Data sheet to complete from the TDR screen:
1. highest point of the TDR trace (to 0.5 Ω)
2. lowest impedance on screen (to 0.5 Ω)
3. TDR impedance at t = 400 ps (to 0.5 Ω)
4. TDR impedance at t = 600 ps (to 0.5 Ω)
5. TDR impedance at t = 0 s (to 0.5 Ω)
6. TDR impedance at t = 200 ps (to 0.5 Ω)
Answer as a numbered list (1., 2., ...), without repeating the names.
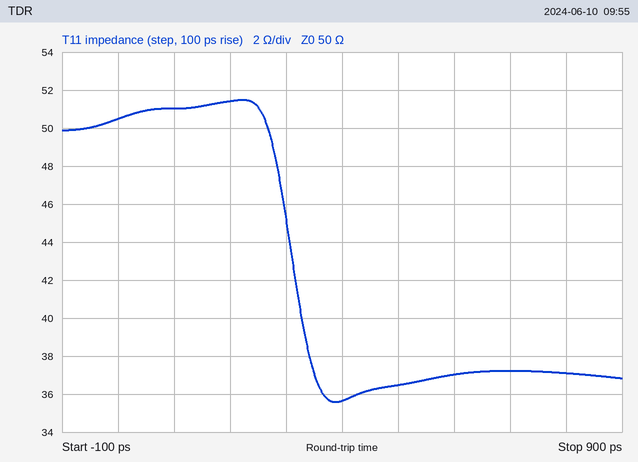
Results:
1. 51.5 Ω
2. 35.5 Ω
3. 35.5 Ω
4. 37.0 Ω
5. 50.5 Ω
6. 51.5 Ω
